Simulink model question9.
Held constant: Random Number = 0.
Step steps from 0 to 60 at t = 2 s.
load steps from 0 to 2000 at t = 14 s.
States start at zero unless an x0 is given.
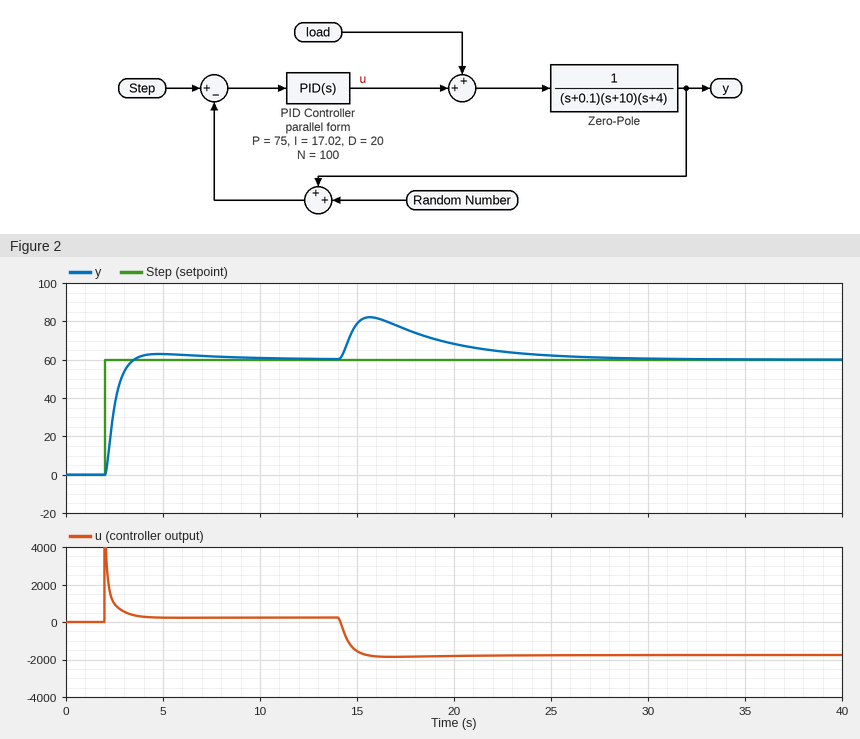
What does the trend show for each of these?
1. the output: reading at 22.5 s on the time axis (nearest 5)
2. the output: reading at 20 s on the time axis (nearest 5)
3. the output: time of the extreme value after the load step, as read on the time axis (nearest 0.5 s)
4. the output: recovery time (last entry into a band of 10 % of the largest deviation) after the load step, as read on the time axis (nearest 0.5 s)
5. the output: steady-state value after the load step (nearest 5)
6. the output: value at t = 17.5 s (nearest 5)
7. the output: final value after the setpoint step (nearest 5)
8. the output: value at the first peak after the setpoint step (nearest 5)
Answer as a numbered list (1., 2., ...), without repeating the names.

1. 65
2. 70
3. 15.5 s
4. 25.0 s
5. 60
6. 75
7. 60
8. 65
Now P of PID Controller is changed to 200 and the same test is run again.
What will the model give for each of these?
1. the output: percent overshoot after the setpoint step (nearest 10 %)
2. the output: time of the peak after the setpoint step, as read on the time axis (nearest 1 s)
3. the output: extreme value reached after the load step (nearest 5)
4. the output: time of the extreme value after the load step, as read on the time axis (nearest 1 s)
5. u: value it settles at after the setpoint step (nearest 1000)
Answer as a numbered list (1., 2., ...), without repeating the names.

1. 20 %
2. 3 s
3. 70
4. 15 s
5. 0
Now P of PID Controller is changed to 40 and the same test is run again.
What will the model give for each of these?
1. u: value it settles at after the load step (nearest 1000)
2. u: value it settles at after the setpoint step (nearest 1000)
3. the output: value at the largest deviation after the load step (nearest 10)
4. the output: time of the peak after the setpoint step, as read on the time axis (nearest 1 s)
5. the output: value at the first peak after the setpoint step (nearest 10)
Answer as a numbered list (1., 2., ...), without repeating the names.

1. -2000
2. 0
3. 90
4. 6 s
5. 70
